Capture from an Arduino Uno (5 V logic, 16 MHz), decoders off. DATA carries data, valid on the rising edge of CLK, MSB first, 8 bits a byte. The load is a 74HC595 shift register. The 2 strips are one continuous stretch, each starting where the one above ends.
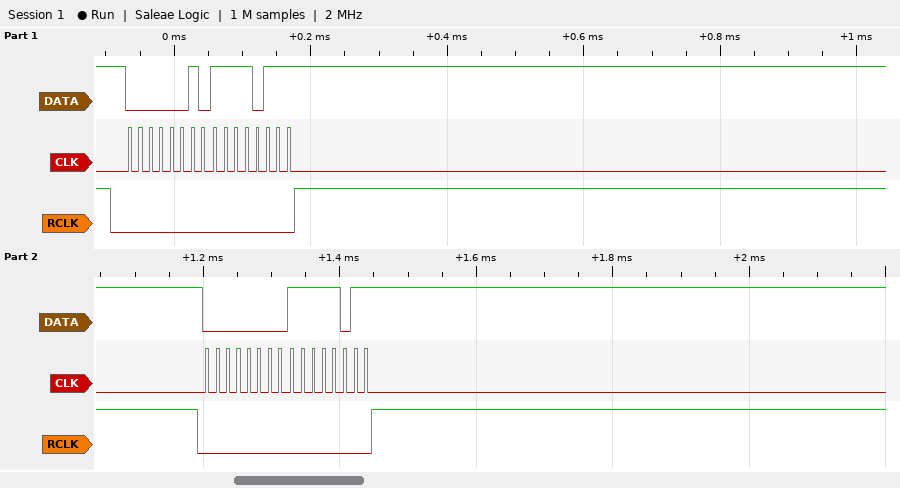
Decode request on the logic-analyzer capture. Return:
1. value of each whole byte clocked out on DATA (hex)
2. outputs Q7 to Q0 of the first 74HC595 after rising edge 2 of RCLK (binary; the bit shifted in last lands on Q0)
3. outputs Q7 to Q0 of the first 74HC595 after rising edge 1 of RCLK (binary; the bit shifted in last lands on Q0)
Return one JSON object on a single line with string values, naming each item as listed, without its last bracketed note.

{"value of each whole byte clocked out on DATA": "0x02 0xF7 0x00 0xFB", "outputs Q7 to Q0 of the first 74HC595 after rising edge 2 of RCLK": "11111011", "outputs Q7 to Q0 of the first 74HC595 after rising edge 1 of RCLK": "11110111"}
